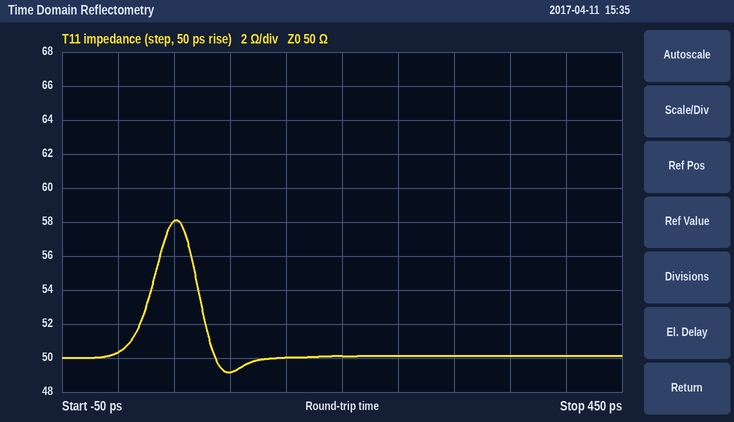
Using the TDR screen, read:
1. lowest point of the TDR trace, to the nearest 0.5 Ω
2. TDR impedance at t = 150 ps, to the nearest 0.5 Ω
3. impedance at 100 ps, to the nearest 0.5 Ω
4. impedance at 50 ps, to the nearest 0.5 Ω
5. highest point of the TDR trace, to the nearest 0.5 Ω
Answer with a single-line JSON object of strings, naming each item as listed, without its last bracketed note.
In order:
{"lowest point of the TDR trace, to the nearest 0.5 Ω": "49.0 Ω", "TDR impedance at t = 150 ps, to the nearest 0.5 Ω": "50.0 Ω", "impedance at 100 ps, to the nearest 0.5 Ω": "49.0 Ω", "impedance at 50 ps, to the nearest 0.5 Ω": "58.0 Ω", "highest point of the TDR trace, to the nearest 0.5 Ω": "58.0 Ω"}
